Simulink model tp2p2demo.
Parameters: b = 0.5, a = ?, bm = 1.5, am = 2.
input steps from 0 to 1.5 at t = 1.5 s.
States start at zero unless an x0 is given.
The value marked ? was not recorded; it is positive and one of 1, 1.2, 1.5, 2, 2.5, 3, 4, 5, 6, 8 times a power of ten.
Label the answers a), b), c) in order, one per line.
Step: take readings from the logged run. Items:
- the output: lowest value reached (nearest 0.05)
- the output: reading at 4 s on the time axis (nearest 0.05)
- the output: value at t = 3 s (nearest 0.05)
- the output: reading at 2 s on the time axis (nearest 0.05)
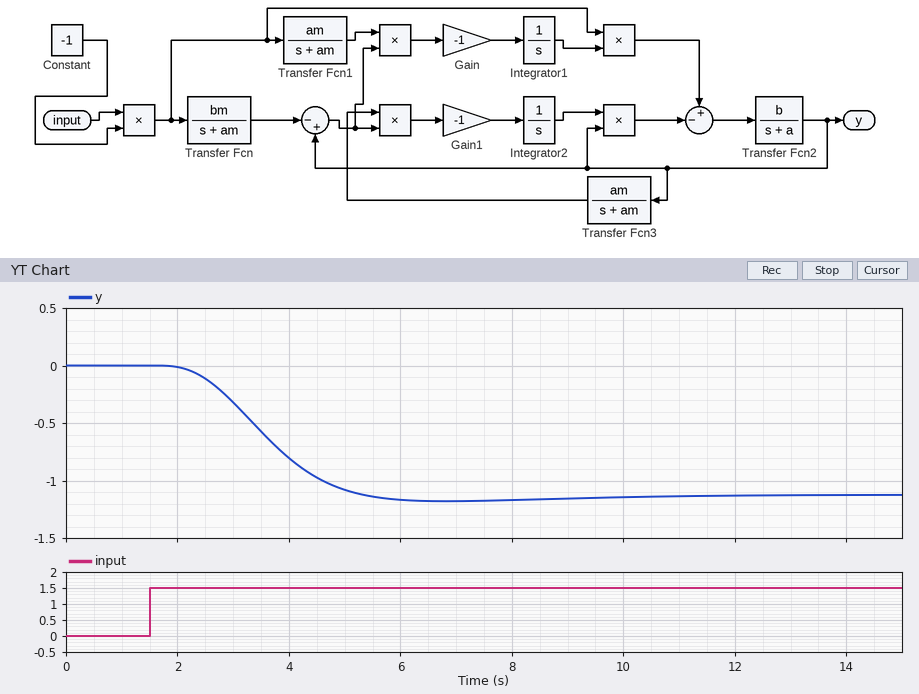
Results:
a) -1.20
b) -0.80
c) -0.30
d) 0.00
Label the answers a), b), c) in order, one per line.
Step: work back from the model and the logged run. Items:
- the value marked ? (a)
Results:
a) 1.2
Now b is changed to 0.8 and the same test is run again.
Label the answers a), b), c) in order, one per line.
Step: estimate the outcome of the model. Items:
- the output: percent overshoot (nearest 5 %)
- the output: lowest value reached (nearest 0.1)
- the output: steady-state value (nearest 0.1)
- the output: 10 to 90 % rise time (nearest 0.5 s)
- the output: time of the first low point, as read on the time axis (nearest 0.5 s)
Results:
a) 15 %
b) -1.3
c) -1.1
d) 1.5 s
e) 5.5 s
